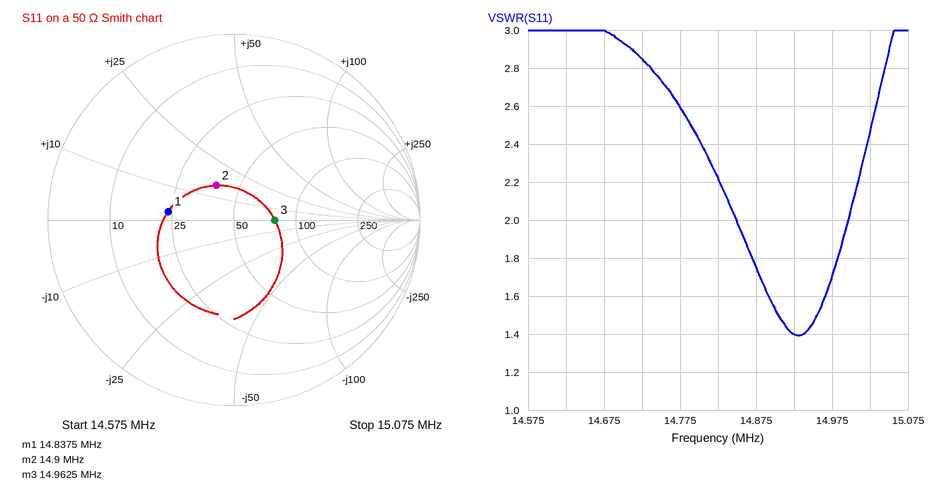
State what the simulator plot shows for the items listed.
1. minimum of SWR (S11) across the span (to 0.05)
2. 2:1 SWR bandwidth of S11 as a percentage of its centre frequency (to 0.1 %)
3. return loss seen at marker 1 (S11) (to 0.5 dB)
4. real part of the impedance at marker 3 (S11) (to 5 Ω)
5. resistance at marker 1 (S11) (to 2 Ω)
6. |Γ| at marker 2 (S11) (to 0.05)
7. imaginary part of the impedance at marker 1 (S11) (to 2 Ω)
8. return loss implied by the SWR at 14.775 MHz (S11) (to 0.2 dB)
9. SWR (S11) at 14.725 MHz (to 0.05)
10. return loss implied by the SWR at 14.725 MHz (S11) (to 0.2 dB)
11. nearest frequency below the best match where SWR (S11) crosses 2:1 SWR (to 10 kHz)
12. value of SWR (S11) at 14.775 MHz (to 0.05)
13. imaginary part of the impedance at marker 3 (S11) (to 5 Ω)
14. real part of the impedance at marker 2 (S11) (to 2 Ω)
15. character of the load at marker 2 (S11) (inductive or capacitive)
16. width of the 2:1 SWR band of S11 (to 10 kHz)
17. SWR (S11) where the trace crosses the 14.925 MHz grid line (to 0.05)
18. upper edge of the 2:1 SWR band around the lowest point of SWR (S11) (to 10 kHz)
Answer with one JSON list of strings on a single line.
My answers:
["1.40", "1.0 %", "9.0 dB", "80 Ω", "24 Ω", "0.20", "+2 Ω", "7.0 dB", "2.85", "6.4 dB", "14.85 MHz", "2.60", "0 Ω", "38 Ω", "inductive", "150 kHz", "1.40", "15.00 MHz"]
